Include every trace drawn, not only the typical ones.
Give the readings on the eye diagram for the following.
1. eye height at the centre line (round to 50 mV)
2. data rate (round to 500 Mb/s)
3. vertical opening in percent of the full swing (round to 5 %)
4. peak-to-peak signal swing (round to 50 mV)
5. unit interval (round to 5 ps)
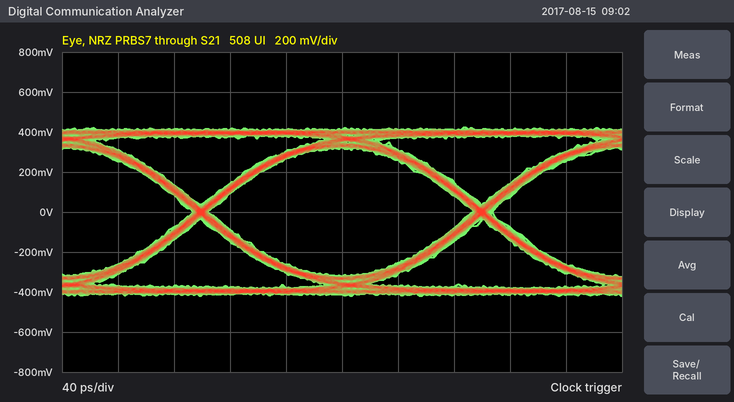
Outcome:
650 mV
5.0 Gb/s
75 %
850 mV
200 ps
